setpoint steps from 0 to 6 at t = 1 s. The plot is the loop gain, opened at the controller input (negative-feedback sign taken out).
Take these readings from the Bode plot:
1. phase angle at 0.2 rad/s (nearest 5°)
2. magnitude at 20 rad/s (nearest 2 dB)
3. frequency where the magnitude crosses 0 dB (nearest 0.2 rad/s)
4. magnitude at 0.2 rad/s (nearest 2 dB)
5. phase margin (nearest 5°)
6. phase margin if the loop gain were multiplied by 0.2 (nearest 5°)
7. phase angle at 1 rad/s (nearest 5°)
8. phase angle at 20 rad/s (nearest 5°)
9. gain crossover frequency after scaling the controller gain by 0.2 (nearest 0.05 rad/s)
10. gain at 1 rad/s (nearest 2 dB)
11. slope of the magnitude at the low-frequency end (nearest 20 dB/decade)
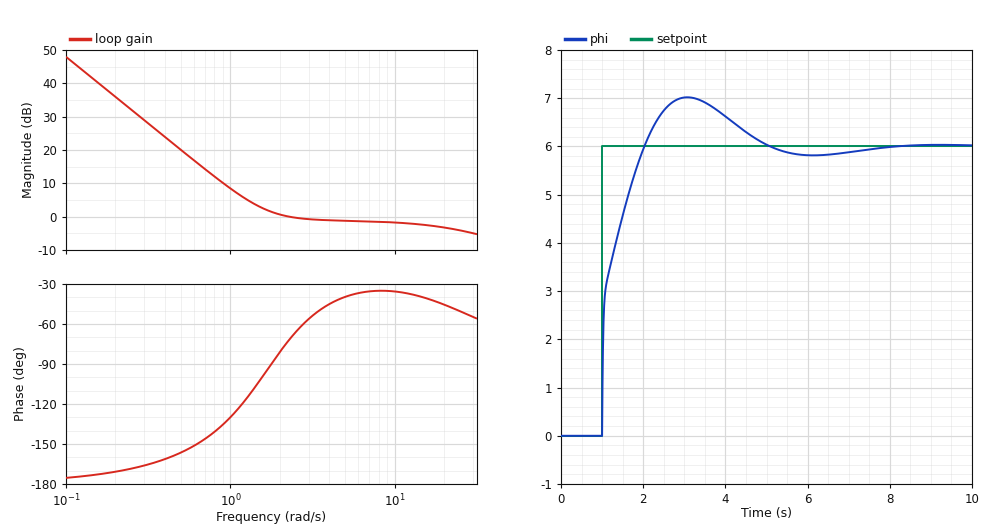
-170°
-4 dB
2.2 rad/s
36 dB
110°
35°
-130°
-45°
0.70 rad/s
8 dB
-40 dB/decade
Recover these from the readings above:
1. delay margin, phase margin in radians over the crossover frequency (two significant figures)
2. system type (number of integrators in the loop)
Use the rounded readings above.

0.87 s
2
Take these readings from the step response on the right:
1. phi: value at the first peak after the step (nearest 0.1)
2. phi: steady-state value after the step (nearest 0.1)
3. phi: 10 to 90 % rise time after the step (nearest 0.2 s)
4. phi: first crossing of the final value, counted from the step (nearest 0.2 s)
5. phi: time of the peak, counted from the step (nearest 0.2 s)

7.0
6.0
0.8 s
1.0 s
2.0 s
